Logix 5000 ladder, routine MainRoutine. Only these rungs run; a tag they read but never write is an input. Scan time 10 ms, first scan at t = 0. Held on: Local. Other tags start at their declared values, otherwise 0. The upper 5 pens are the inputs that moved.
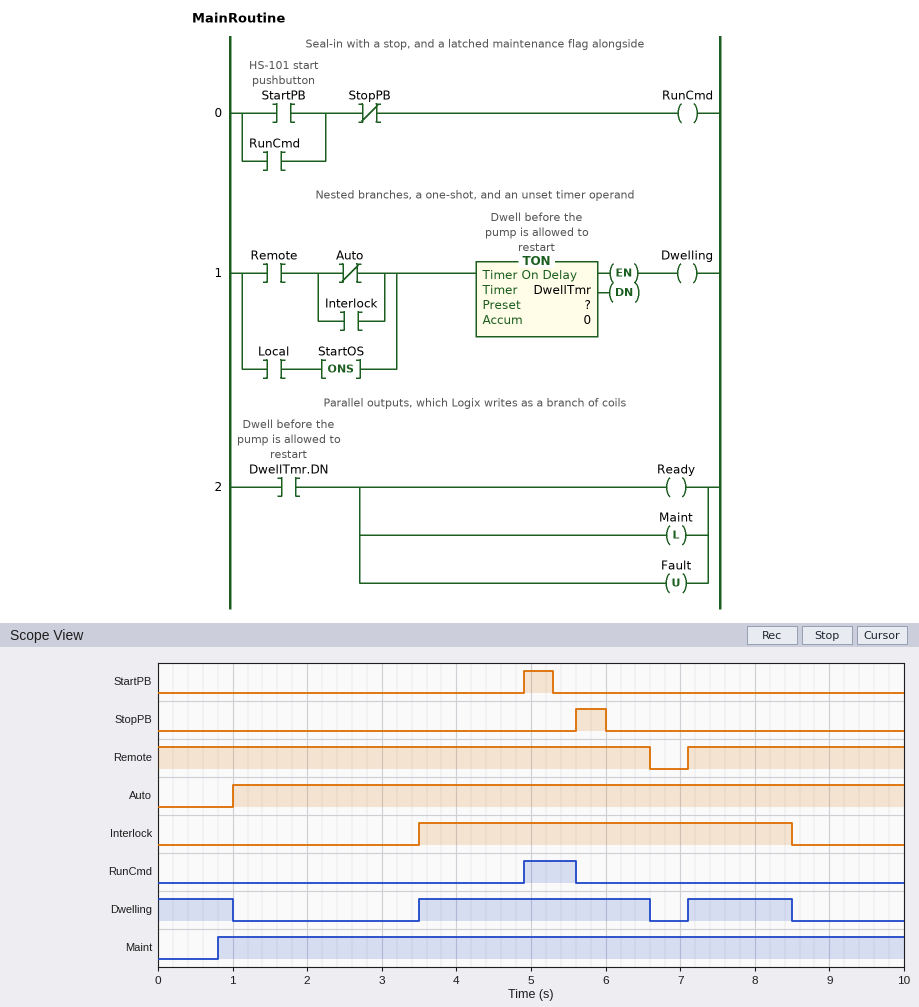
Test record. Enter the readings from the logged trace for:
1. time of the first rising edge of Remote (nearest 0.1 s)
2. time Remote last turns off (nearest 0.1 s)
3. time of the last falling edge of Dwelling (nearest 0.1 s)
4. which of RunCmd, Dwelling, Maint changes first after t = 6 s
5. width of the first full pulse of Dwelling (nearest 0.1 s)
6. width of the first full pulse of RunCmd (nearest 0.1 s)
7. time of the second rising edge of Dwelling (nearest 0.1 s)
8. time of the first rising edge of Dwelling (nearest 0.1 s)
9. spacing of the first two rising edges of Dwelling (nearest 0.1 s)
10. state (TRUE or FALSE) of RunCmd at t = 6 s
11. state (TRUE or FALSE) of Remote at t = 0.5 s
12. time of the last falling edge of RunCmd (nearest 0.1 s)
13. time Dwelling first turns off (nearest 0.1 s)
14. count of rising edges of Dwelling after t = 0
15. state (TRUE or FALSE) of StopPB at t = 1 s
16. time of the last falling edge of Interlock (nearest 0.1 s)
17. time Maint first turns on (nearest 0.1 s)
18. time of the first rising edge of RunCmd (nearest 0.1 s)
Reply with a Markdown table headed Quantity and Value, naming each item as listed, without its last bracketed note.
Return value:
| Quantity | Value |
|---|---|
| time of the first rising edge of Remote | 7.1 s |
| time Remote last turns off | 6.6 s |
| time of the last falling edge of Dwelling | 8.5 s |
| which of RunCmd, Dwelling, Maint changes first after t = 6 s | Dwelling |
| width of the first full pulse of Dwelling | 3.1 s |
| width of the first full pulse of RunCmd | 0.7 s |
| time of the second rising edge of Dwelling | 7.1 s |
| time of the first rising edge of Dwelling | 3.5 s |
| spacing of the first two rising edges of Dwelling | 3.6 s |
| state (TRUE or FALSE) of RunCmd at t = 6 s | FALSE |
| state (TRUE or FALSE) of Remote at t = 0.5 s | TRUE |
| time of the last falling edge of RunCmd | 5.6 s |
| time Dwelling first turns off | 1.0 s |
| count of rising edges of Dwelling after t = 0 | 2 |
| state (TRUE or FALSE) of StopPB at t = 1 s | FALSE |
| time of the last falling edge of Interlock | 8.5 s |
| time Maint first turns on | 0.8 s |
| time of the first rising edge of RunCmd | 4.9 s |
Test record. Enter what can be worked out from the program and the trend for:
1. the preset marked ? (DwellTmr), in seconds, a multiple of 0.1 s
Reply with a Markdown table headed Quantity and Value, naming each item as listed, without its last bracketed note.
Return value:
| Quantity | Value |
|---|---|
| the preset marked ? (DwellTmr), in seconds, a multiple of 0.1 s | 0.8 s |
